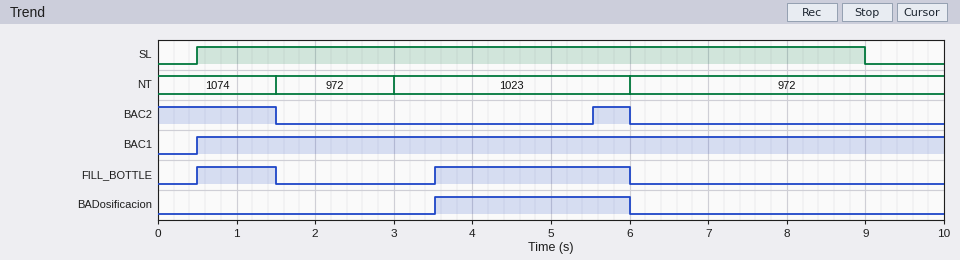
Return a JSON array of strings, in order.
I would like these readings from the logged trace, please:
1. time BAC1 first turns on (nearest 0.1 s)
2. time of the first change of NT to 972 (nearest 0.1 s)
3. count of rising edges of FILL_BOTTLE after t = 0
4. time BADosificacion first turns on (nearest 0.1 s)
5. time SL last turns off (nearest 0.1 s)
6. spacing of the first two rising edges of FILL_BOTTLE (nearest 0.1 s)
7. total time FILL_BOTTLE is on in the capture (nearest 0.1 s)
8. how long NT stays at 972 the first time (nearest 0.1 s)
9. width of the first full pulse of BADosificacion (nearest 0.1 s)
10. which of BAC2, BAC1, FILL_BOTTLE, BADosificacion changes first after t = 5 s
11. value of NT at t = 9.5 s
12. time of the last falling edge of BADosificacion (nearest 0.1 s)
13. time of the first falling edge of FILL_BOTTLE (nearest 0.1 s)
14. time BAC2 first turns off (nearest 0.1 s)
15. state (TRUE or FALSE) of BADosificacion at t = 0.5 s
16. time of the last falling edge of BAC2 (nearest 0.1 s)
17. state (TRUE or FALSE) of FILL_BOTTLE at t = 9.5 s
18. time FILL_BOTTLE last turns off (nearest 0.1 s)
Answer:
["0.5 s", "1.5 s", "2", "3.5 s", "9.0 s", "3.0 s", "3.5 s", "1.5 s", "2.5 s", "BAC2", "972", "6.0 s", "1.5 s", "1.5 s", "FALSE", "6.0 s", "FALSE", "6.0 s"]
